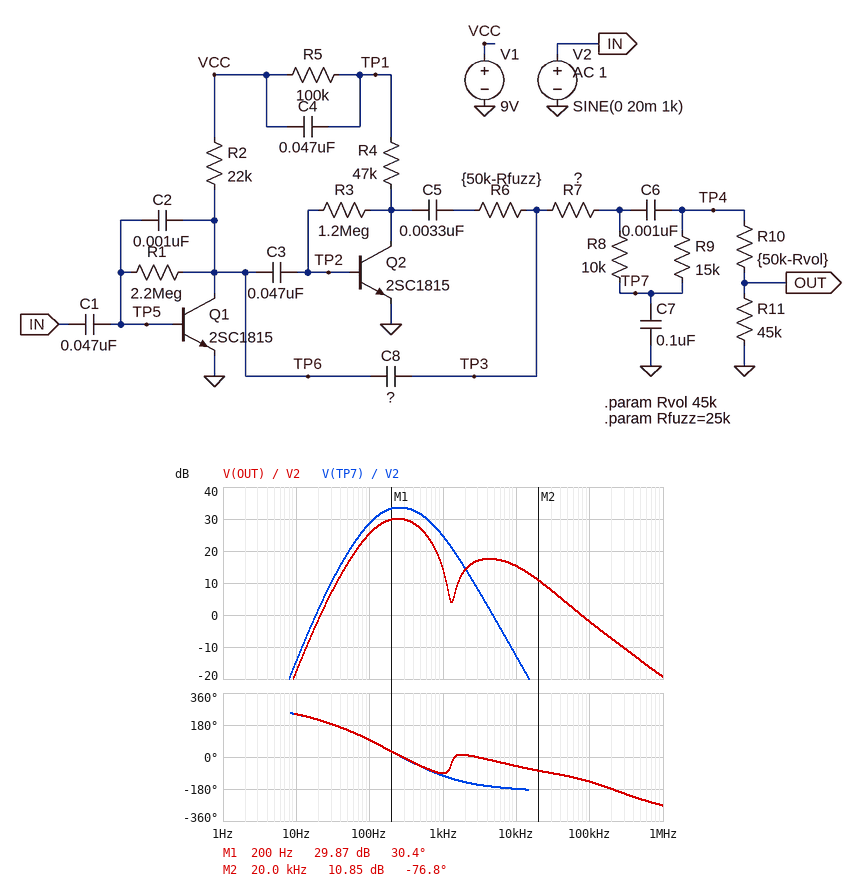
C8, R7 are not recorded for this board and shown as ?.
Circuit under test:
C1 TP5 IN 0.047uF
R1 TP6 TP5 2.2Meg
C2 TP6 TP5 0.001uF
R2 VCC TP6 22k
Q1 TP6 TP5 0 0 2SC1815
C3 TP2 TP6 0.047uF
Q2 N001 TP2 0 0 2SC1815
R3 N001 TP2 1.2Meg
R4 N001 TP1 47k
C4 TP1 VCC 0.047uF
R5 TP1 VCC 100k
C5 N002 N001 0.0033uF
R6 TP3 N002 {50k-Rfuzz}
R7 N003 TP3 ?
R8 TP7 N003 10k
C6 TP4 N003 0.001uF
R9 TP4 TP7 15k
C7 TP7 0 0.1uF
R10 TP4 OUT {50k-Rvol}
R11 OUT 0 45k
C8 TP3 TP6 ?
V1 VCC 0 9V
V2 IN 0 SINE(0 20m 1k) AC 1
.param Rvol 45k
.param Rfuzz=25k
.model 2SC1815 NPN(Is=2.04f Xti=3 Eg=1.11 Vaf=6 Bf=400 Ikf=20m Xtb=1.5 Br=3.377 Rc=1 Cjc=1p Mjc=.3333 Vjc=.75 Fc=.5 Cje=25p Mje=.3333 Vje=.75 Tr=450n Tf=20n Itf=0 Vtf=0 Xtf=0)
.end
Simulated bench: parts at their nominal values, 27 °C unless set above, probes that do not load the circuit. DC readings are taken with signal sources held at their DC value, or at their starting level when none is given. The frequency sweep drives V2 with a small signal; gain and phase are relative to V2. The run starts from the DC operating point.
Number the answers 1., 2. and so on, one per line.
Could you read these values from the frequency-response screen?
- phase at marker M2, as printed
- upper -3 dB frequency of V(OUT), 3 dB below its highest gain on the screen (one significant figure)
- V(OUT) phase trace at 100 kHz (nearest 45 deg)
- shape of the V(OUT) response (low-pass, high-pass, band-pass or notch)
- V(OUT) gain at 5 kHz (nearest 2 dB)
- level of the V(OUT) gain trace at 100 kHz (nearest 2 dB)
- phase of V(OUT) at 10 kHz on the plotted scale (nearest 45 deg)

1. -76.8 deg
2. 500 Hz
3. -135 deg
4. band-pass
5. 18 dB
6. -2 dB
7. -45 deg
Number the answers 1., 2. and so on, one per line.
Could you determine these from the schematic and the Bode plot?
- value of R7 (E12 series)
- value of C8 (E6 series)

1. 82 kΩ
2. 1 nF
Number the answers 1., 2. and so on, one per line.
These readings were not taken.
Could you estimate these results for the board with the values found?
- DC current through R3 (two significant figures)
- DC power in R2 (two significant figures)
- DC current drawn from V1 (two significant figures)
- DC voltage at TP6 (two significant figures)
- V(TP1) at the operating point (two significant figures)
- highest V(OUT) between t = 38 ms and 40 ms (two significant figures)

1. 140 nA
2. 2.2 mW
3. 370 µA
4. 2.1 V
5. 3.4 V
6. 18 mV
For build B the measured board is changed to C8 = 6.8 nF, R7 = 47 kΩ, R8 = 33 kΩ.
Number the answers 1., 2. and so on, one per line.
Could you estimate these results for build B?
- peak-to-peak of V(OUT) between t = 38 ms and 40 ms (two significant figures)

1. 45 mV
